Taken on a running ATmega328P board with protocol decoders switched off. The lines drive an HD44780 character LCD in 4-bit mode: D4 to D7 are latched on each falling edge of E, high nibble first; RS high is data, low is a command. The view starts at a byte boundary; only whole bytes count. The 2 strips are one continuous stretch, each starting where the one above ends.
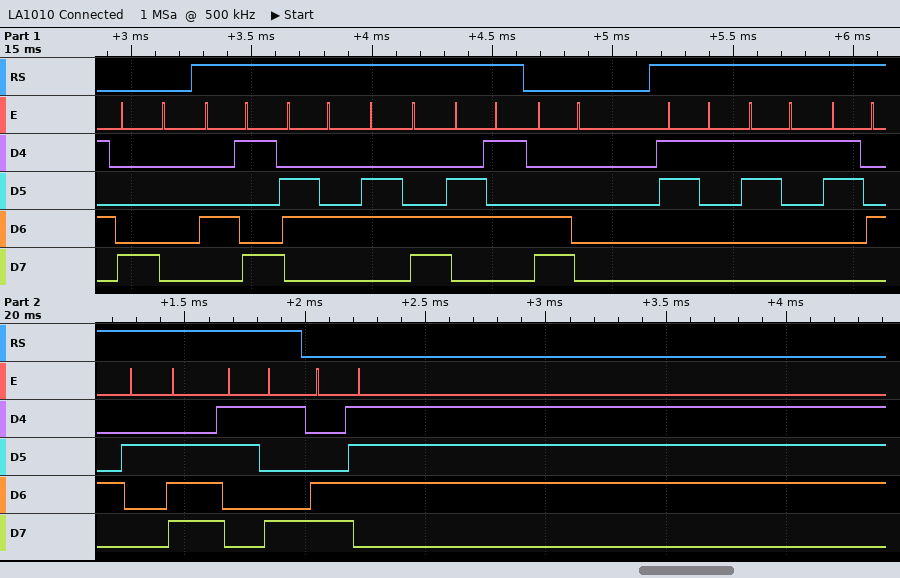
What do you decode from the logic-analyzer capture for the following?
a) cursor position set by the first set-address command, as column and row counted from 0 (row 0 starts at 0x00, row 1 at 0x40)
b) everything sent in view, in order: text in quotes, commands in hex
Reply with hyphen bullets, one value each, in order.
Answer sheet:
- column 0, row 0
- 0x80 "Idle" 0xC0 "114.9" 0xC7
